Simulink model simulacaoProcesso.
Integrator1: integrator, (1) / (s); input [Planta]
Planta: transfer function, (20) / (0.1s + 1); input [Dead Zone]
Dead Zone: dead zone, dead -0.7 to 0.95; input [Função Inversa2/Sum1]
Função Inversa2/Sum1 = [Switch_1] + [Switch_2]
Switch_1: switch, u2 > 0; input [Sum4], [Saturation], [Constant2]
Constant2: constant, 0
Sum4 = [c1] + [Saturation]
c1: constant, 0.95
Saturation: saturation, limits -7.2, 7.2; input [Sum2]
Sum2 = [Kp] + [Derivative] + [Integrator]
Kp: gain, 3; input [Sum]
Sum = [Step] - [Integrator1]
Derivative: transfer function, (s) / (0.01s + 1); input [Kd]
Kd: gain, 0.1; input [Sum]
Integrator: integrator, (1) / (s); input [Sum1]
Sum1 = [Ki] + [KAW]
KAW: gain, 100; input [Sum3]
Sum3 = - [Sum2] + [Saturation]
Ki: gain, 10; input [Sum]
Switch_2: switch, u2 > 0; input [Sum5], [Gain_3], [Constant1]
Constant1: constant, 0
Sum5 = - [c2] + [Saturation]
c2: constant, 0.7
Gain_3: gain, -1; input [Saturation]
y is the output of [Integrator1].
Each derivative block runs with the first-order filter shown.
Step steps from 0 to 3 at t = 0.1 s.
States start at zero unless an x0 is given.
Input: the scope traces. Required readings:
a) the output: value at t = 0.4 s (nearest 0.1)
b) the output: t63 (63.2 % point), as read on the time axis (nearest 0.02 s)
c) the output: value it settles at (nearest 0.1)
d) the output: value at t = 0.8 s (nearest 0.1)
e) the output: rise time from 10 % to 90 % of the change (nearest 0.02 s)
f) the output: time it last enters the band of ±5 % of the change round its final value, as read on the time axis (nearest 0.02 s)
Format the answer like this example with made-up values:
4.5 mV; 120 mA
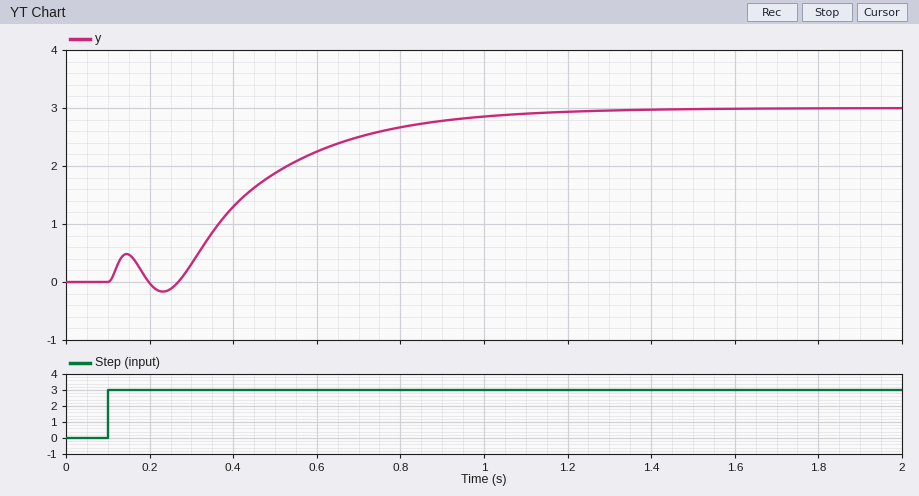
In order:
1.3; 0.50 s; 3.0; 2.7; 0.70 s; 1.00 s
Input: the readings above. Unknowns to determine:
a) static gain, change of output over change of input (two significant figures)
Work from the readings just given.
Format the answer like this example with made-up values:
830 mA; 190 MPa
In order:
1.0
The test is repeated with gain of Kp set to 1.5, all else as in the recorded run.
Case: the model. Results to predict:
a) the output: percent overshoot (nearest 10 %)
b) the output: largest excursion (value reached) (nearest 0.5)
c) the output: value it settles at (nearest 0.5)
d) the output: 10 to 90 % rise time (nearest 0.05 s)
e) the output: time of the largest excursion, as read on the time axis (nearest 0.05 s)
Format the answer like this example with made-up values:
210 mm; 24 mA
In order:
20 %; 3.5; 3.0; 0.35 s; 0.65 s
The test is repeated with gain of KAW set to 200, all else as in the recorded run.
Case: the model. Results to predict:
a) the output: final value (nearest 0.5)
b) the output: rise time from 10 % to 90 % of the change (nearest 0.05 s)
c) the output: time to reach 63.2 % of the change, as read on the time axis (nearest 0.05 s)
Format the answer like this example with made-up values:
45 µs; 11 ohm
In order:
3.0; 0.55 s; 0.60 s
